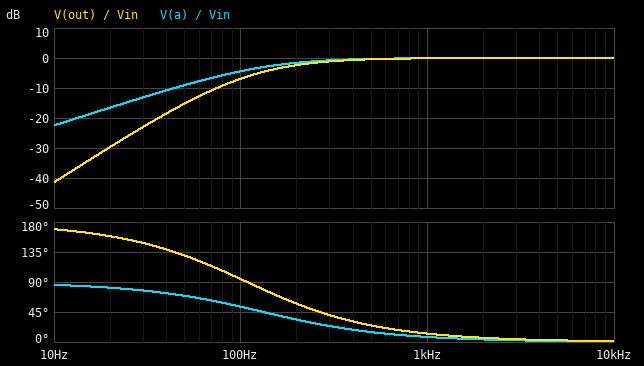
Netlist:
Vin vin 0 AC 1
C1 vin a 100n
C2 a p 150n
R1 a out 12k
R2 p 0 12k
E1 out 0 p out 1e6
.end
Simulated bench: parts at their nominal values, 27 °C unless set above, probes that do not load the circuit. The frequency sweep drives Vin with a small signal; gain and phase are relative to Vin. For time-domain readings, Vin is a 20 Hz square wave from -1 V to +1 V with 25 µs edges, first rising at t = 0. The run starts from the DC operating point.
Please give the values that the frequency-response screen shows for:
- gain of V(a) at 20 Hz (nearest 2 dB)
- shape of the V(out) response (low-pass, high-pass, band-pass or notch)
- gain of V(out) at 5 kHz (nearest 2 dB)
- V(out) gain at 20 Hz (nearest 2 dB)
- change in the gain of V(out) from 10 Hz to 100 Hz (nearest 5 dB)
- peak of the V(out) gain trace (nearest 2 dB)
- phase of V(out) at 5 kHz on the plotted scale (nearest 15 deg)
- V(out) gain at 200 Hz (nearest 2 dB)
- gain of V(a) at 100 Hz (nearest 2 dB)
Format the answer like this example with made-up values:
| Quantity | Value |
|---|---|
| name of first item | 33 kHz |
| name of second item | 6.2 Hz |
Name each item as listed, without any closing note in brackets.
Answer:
| Quantity | Value |
|---|---|
| gain of V(a) at 20 Hz | -16 dB |
| shape of the V(out) response | high-pass |
| gain of V(out) at 5 kHz | 0 dB |
| V(out) gain at 20 Hz | -30 dB |
| change in the gain of V(out) from 10 Hz to 100 Hz | 35 dB |
| peak of the V(out) gain trace | 0 dB |
| phase of V(out) at 5 kHz on the plotted scale | 0 deg |
| V(out) gain at 200 Hz | -2 dB |
| gain of V(a) at 100 Hz | -4 dB |
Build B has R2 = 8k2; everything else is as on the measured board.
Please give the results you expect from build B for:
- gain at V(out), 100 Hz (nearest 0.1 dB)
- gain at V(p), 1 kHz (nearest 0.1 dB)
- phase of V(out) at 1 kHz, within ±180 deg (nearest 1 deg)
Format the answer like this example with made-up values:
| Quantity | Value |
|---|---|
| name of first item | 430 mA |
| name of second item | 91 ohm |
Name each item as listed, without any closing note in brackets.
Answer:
| Quantity | Value |
|---|---|
| gain at V(out), 100 Hz | -10.4 dB |
| gain at V(p), 1 kHz | -0.3 dB |
| phase of V(out) at 1 kHz, within ±180 deg | 18 deg |
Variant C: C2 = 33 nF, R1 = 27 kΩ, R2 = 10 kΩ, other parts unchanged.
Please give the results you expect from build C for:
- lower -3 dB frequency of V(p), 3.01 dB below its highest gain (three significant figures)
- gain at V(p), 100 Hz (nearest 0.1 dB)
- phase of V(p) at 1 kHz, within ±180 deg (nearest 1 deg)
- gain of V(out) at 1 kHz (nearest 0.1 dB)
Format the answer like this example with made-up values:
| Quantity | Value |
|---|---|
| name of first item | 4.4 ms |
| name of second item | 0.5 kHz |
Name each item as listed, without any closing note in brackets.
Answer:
| Quantity | Value |
|---|---|
| lower -3 dB frequency of V(p), 3.01 dB below its highest gain | 597 Hz |
| gain at V(p), 100 Hz | -16.5 dB |
| phase of V(p) at 1 kHz, within ±180 deg | 33 deg |
| gain of V(out) at 1 kHz | -1.3 dB |
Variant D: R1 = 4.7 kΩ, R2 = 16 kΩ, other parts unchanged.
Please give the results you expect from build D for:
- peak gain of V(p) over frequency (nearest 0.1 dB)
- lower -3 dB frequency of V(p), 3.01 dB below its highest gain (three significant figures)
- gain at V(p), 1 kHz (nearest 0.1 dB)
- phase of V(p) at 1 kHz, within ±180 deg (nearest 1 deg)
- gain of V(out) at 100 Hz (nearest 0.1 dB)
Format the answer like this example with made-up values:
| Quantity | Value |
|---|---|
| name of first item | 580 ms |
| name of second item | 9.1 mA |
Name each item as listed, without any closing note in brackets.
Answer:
| Quantity | Value |
|---|---|
| peak gain of V(p) over frequency | 0.7 dB |
| lower -3 dB frequency of V(p), 3.01 dB below its highest gain | 131 Hz |
| gain at V(p), 1 kHz | 0.1 dB |
| phase of V(p) at 1 kHz, within ±180 deg | 10 deg |
| gain of V(out) at 100 Hz | -6.3 dB |
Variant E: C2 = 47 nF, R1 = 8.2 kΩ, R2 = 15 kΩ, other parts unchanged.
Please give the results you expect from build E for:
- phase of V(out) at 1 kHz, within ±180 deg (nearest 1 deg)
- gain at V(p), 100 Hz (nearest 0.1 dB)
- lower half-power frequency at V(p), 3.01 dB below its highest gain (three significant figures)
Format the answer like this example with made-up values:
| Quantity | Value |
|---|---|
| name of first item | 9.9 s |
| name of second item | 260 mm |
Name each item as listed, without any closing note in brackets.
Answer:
| Quantity | Value |
|---|---|
| phase of V(out) at 1 kHz, within ±180 deg | 19 deg |
| gain at V(p), 100 Hz | -13.5 dB |
| lower half-power frequency at V(p), 3.01 dB below its highest gain | 238 Hz |
